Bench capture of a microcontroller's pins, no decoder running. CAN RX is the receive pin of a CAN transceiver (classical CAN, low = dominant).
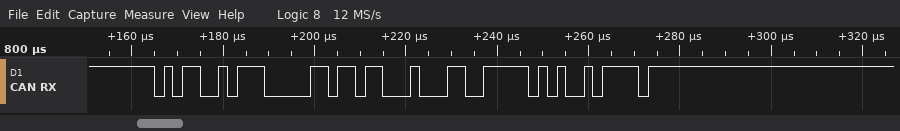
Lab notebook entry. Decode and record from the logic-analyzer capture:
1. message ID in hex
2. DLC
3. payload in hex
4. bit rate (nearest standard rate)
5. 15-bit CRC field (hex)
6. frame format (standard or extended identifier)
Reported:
0x597
2
D8 8C
500 kbit/s
0x7E97
standard
